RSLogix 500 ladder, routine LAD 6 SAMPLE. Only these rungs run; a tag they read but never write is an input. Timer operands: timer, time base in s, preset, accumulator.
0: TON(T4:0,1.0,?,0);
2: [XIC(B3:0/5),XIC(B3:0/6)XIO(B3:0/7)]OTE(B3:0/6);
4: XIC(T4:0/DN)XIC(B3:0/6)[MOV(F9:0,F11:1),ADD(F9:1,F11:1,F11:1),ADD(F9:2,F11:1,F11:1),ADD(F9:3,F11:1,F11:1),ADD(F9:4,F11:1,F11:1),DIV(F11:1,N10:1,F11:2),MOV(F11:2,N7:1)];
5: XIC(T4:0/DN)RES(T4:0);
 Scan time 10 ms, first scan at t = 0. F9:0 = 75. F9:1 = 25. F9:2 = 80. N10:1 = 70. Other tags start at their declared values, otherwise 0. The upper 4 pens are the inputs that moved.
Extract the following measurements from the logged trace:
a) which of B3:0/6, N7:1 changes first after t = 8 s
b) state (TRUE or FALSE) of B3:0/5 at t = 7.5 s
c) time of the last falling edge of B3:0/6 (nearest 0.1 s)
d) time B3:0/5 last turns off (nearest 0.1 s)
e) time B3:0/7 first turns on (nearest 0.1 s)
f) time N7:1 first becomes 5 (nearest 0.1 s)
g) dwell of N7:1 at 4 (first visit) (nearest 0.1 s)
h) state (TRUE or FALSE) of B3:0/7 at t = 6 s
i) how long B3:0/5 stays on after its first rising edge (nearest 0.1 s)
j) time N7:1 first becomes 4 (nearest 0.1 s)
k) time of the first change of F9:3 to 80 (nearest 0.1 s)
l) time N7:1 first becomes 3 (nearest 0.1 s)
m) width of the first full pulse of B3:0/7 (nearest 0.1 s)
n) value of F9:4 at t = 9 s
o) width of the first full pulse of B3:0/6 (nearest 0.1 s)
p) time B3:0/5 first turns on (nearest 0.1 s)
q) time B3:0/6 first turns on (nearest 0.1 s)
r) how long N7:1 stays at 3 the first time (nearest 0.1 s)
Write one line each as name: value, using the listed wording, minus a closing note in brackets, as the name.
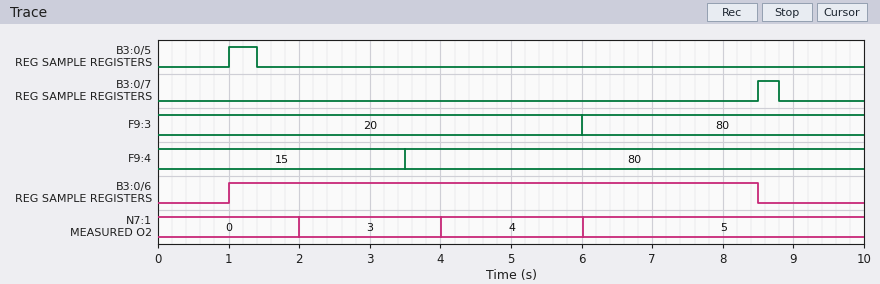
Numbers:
which of B3:0/6, N7:1 changes first after t = 8 s: B3:0/6
state (TRUE or FALSE) of B3:0/5 at t = 7.5 s: FALSE
time of the last falling edge of B3:0/6: 8.5 s
time B3:0/5 last turns off: 1.4 s
time B3:0/7 first turns on: 8.5 s
time N7:1 first becomes 5: 6.0 s
dwell of N7:1 at 4 (first visit): 2.0 s
state (TRUE or FALSE) of B3:0/7 at t = 6 s: FALSE
how long B3:0/5 stays on after its first rising edge: 0.4 s
time N7:1 first becomes 4: 4.0 s
time of the first change of F9:3 to 80: 6.0 s
time N7:1 first becomes 3: 2.0 s
width of the first full pulse of B3:0/7: 0.3 s
value of F9:4 at t = 9 s: 80
width of the first full pulse of B3:0/6: 7.5 s
time B3:0/5 first turns on: 1.0 s
time B3:0/6 first turns on: 1.0 s
how long N7:1 stays at 3 the first time: 2.0 s
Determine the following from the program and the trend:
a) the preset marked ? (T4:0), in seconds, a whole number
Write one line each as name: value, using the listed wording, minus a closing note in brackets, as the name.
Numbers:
the preset marked ? (T4:0), in seconds, a whole number: 2 s
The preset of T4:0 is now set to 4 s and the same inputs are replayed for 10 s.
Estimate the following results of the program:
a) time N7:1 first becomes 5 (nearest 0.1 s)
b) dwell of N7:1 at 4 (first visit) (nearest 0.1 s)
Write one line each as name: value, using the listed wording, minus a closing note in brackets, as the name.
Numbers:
time N7:1 first becomes 5: 8.0 s
dwell of N7:1 at 4 (first visit): 4.0 s
